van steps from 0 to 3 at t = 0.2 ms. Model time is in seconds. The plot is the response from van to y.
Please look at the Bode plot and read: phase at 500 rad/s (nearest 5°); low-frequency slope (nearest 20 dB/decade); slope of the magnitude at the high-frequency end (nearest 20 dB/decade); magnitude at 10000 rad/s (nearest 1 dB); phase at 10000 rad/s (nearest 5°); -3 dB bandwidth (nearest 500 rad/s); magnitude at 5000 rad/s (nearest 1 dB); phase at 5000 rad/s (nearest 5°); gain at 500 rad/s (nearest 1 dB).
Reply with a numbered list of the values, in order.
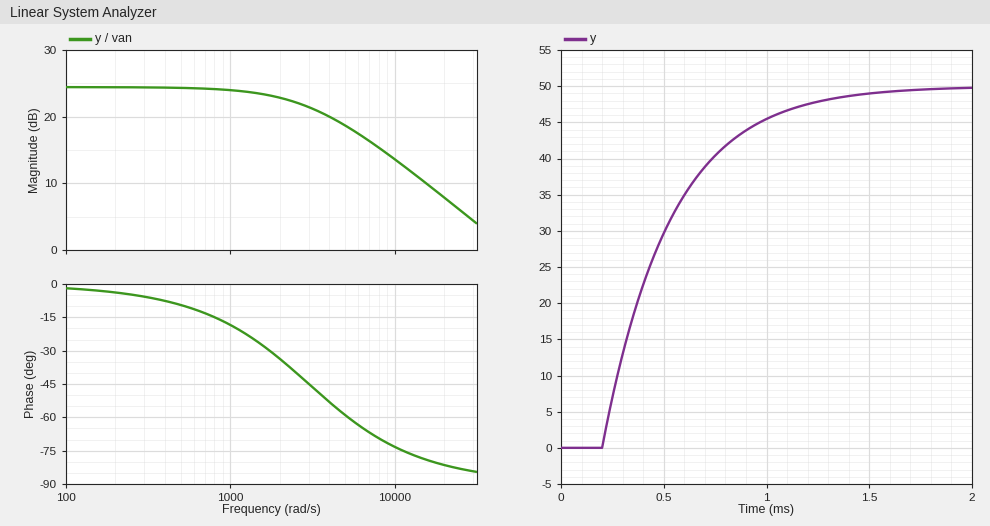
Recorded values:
1. -10°
2. 0 dB/decade
3. -20 dB/decade
4. 14 dB
5. -75°
6. 3000 rad/s
7. 19 dB
8. -60°
9. 24 dB
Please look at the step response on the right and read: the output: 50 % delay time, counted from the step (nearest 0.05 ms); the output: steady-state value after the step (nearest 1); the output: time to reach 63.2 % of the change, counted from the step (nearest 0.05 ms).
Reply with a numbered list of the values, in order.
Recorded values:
1. 0.25 ms
2. 50
3. 0.35 ms
